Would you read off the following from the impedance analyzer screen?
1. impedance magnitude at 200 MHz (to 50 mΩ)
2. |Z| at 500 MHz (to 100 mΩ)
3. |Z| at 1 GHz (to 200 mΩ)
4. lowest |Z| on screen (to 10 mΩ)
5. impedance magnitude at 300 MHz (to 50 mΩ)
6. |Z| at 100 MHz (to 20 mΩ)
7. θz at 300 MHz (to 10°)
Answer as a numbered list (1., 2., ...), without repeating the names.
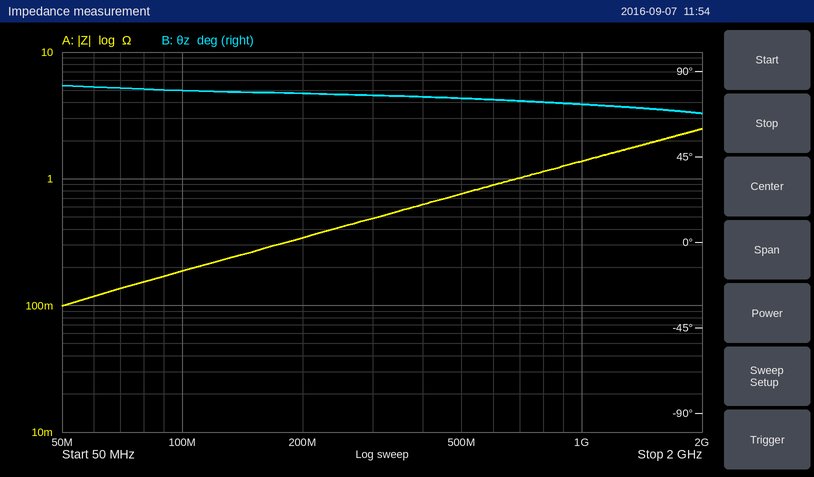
1. 350 mΩ
2. 800 mΩ
3. 1.4 Ω
4. 100 mΩ
5. 500 mΩ
6. 180 mΩ
7. 80°
